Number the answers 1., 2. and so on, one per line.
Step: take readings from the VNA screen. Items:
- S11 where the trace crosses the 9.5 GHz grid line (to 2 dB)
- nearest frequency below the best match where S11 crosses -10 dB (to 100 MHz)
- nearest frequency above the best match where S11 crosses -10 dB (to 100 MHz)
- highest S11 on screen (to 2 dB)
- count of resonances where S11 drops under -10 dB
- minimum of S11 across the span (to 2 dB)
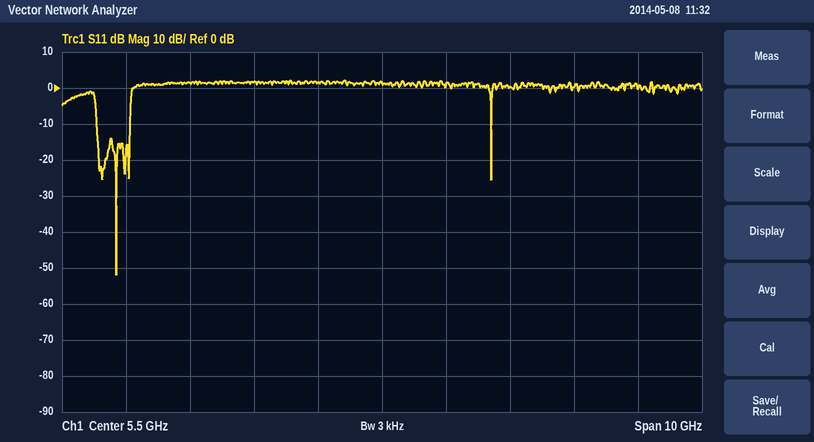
1. 0 dB
2. 1.0 GHz
3. 1.6 GHz
4. 2 dB
5. 5
6. -52 dB
